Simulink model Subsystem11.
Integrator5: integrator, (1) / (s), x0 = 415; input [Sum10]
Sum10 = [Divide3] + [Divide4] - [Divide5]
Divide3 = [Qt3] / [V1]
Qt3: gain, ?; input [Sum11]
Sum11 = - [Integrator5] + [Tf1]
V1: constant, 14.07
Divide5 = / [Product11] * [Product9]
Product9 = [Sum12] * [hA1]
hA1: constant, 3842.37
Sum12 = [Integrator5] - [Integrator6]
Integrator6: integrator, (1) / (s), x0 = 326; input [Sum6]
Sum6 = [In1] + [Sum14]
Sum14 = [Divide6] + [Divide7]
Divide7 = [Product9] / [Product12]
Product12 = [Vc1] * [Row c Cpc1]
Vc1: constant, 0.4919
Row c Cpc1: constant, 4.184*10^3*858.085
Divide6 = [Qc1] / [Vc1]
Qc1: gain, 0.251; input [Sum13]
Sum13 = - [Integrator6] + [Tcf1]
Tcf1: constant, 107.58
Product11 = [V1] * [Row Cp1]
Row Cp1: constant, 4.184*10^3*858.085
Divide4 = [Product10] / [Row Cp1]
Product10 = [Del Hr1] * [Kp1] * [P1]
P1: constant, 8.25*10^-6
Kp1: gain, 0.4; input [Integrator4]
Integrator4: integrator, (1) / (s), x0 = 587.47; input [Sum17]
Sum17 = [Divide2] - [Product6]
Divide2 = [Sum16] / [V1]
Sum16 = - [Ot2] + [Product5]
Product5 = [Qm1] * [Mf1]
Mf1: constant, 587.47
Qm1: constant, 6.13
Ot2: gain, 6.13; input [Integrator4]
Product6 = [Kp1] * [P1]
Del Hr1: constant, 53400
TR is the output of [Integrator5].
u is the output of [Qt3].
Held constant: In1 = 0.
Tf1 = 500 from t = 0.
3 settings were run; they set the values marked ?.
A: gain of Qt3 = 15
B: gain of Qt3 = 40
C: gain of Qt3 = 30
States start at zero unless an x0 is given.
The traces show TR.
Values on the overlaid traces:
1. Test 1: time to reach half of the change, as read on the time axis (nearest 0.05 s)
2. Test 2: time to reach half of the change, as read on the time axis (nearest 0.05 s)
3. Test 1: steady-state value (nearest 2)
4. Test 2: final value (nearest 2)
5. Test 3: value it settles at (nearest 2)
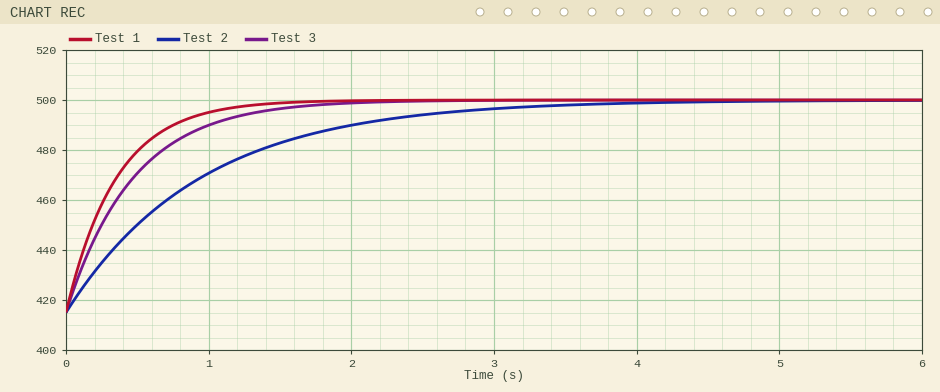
0.25 s
0.65 s
500
500
500
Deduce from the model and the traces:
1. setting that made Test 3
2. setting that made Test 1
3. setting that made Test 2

C
B
A
